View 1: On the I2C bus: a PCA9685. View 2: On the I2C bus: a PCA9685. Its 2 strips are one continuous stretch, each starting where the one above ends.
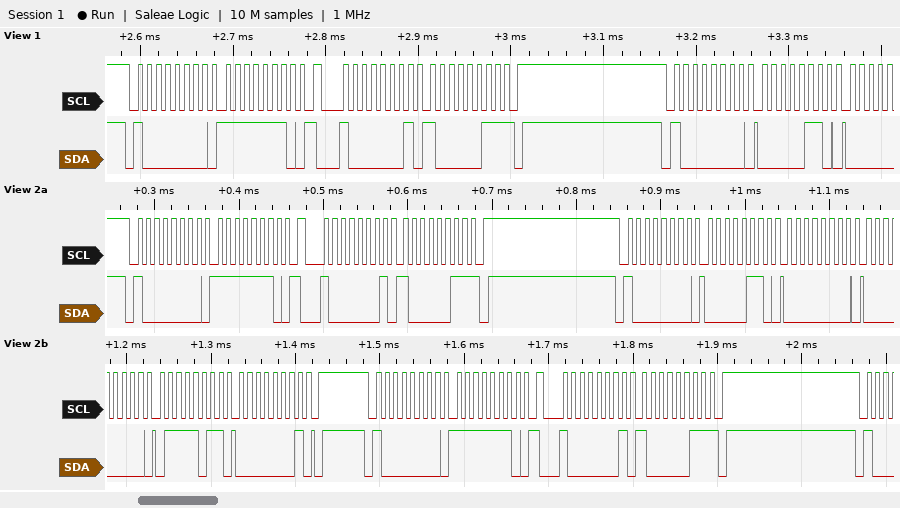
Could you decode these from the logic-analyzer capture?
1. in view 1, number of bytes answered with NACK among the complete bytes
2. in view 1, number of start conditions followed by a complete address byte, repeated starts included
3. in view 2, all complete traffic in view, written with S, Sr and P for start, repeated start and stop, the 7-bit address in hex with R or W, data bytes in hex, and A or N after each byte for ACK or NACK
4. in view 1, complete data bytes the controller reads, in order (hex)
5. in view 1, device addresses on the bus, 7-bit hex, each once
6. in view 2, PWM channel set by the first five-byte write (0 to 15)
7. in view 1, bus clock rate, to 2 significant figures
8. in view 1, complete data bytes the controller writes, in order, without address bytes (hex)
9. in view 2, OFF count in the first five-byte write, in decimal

1
3
S 40W A FE A Sr 40R A 83 N P S 40W A 06 A 00 A 00 A 7B A 01 A P S 40W A FE A Sr 40R A 83 N P
83
0x40
0
100 kHz
FE 06
379
